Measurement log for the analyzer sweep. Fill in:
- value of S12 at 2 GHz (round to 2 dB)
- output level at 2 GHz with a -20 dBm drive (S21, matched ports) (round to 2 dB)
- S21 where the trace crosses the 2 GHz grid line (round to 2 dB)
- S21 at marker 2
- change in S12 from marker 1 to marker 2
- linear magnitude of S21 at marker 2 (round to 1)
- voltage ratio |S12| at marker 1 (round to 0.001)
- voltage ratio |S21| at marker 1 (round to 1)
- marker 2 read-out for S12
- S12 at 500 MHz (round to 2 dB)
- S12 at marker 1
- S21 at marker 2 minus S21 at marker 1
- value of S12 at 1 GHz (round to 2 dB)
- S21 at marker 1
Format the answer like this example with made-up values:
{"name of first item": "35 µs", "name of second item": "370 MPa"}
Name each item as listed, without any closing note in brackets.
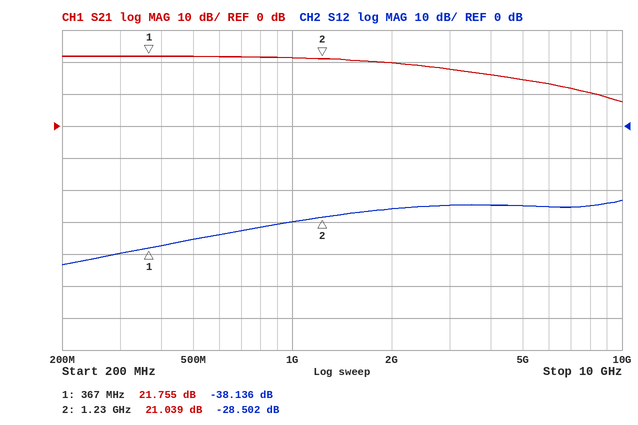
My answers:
{"value of S12 at 2 GHz": "-26 dB", "output level at 2 GHz with a -20 dBm drive (S21, matched ports)": "0 dBm", "S21 where the trace crosses the 2 GHz grid line": "20 dB", "S21 at marker 2": "21.039 dB", "change in S12 from marker 1 to marker 2": "9.634 dB", "linear magnitude of S21 at marker 2": "11", "voltage ratio |S12| at marker 1": "0.012", "voltage ratio |S21| at marker 1": "12", "marker 2 read-out for S12": "-28.502 dB", "S12 at 500 MHz": "-36 dB", "S12 at marker 1": "-38.136 dB", "S21 at marker 2 minus S21 at marker 1": "-0.716 dB", "value of S12 at 1 GHz": "-30 dB", "S21 at marker 1": "21.755 dB"}
